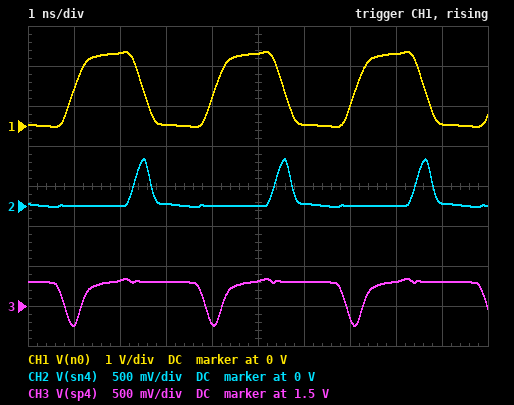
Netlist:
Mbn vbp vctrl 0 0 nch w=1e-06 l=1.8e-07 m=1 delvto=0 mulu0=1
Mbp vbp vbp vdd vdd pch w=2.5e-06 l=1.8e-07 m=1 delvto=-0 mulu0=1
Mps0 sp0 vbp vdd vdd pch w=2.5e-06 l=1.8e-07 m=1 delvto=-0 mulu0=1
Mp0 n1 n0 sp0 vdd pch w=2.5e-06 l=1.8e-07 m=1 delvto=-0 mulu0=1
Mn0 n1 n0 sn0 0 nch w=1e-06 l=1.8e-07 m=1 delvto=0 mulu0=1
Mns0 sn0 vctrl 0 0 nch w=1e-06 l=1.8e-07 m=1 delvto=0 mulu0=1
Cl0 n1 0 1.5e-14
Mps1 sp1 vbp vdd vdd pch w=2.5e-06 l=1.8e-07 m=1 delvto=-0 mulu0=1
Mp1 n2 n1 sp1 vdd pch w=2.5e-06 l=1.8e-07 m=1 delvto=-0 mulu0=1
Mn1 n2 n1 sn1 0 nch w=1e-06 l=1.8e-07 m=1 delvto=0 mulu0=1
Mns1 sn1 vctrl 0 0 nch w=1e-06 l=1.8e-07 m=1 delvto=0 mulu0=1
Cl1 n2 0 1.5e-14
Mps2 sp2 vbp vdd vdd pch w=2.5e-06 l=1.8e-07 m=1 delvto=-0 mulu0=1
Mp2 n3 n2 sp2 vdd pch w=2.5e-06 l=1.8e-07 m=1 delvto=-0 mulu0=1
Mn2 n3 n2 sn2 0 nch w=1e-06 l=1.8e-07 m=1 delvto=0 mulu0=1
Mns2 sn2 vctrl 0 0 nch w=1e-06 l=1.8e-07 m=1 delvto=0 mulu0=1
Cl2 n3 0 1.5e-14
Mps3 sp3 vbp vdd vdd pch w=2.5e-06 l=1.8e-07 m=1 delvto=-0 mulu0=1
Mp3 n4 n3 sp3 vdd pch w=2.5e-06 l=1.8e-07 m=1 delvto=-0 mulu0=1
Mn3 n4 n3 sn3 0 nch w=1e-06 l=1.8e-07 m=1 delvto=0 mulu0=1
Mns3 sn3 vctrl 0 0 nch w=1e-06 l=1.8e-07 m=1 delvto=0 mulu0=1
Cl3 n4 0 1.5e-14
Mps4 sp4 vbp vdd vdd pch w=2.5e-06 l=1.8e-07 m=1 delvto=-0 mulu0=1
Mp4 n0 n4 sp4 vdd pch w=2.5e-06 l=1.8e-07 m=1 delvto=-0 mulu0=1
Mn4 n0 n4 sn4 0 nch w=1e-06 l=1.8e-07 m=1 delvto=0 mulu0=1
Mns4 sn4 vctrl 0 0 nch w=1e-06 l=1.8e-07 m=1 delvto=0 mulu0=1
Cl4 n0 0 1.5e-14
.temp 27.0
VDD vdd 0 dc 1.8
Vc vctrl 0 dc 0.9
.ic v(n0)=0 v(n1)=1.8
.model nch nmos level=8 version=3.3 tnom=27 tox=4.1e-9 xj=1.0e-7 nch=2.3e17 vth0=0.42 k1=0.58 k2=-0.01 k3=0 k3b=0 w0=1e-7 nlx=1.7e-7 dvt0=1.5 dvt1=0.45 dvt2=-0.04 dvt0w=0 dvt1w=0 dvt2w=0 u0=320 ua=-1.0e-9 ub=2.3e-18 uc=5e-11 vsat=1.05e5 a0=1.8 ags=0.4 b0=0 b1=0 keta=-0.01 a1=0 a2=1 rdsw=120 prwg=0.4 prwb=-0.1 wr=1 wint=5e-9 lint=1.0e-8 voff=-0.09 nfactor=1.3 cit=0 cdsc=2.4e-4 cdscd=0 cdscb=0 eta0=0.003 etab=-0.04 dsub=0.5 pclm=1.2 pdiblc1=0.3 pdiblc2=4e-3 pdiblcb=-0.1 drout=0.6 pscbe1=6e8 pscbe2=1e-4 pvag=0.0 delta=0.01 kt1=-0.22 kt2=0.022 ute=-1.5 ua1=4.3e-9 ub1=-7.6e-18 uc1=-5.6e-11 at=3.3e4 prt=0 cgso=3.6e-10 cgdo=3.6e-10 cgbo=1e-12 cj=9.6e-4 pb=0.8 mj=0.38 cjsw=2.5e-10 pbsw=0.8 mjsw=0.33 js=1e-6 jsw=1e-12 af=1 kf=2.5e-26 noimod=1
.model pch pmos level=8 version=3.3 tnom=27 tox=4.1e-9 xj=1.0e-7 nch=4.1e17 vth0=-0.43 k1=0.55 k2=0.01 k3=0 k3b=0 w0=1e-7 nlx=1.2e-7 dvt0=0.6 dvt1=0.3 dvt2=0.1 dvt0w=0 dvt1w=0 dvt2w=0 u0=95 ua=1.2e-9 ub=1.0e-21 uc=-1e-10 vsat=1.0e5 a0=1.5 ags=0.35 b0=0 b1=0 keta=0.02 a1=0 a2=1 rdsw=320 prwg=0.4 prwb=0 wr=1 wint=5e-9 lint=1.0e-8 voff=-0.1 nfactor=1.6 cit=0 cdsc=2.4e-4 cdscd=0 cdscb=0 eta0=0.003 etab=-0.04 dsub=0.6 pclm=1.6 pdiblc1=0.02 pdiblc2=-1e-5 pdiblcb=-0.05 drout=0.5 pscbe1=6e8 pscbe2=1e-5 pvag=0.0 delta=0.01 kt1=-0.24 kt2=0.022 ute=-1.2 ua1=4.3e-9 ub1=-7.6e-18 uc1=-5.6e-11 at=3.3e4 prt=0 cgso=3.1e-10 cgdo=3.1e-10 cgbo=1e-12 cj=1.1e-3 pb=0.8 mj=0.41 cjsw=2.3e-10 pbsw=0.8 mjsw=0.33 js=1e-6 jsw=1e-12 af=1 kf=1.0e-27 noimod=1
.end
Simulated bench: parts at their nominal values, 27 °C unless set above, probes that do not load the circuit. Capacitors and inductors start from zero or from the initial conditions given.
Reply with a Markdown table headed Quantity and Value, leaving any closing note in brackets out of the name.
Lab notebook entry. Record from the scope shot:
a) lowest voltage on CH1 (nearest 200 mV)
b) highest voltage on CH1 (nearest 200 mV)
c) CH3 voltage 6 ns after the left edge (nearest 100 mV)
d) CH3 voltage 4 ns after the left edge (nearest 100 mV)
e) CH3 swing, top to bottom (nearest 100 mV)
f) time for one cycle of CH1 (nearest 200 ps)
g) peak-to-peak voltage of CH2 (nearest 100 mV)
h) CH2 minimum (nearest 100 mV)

| Quantity | Value |
|---|---|
| lowest voltage on CH1 | 0 V |
| highest voltage on CH1 | 1.8 V |
| CH3 voltage 6 ns after the left edge | 1.8 V |
| CH3 voltage 4 ns after the left edge | 1.3 V |
| CH3 swing, top to bottom | 600 mV |
| time for one cycle of CH1 | 3.0 ns |
| peak-to-peak voltage of CH2 | 600 mV |
| CH2 minimum | 0 V |
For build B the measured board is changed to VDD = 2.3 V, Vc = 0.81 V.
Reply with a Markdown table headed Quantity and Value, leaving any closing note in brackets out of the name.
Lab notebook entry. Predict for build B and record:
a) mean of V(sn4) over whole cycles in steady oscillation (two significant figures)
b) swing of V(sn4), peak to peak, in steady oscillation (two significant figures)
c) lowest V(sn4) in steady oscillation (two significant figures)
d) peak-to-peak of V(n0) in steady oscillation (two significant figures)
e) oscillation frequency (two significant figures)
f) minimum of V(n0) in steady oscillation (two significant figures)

| Quantity | Value |
|---|---|
| mean of V(sn4) over whole cycles in steady oscillation | 140 mV |
| swing of V(sn4), peak to peak, in steady oscillation | 1.1 V |
| lowest V(sn4) in steady oscillation | -15 mV |
| peak-to-peak of V(n0) in steady oscillation | 2.4 V |
| oscillation frequency | 200 MHz |
| minimum of V(n0) in steady oscillation | -18 mV |
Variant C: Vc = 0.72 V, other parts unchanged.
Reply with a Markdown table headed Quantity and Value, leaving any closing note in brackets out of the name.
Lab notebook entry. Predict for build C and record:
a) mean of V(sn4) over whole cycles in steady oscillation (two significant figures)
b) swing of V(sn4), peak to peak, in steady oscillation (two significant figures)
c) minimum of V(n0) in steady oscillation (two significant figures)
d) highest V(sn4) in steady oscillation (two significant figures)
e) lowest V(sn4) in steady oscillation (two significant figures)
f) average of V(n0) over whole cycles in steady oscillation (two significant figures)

| Quantity | Value |
|---|---|
| mean of V(sn4) over whole cycles in steady oscillation | 100 mV |
| swing of V(sn4), peak to peak, in steady oscillation | 790 mV |
| minimum of V(n0) in steady oscillation | -14 mV |
| highest V(sn4) in steady oscillation | 780 mV |
| lowest V(sn4) in steady oscillation | -12 mV |
| average of V(n0) over whole cycles in steady oscillation | 900 mV |
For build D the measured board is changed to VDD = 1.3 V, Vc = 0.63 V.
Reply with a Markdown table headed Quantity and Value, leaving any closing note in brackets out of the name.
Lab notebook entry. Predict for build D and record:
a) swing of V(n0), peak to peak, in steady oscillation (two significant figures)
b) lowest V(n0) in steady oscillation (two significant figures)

| Quantity | Value |
|---|---|
| swing of V(n0), peak to peak, in steady oscillation | 1.3 V |
| lowest V(n0) in steady oscillation | -9.2 mV |
